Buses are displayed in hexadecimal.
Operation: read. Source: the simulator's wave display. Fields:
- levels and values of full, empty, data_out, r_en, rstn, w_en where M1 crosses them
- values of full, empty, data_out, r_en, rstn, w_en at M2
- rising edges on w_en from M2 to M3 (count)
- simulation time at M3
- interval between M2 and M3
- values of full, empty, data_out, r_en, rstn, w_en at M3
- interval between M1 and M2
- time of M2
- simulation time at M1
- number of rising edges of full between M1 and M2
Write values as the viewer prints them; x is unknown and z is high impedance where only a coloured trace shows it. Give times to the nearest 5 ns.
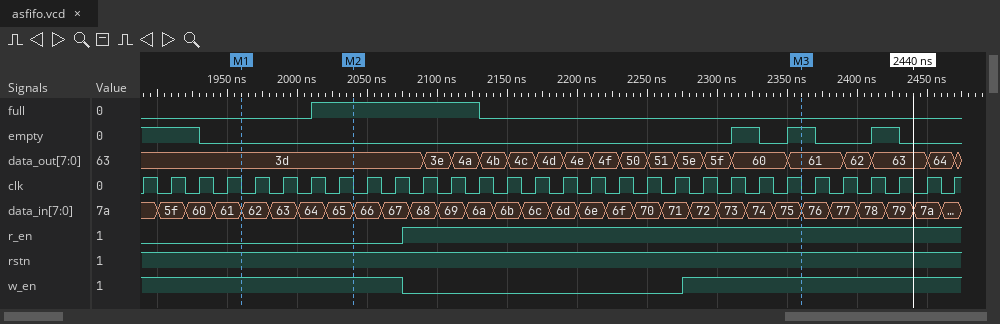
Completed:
full=0, empty=0, data_out=3d, r_en=0, rstn=1, w_en=1
full=1, empty=0, data_out=3d, r_en=0, rstn=1, w_en=1
1
2360 ns
320 ns
full=0, empty=1, data_out=61, r_en=1, rstn=1, w_en=1
80 ns
2040 ns
1960 ns
1
